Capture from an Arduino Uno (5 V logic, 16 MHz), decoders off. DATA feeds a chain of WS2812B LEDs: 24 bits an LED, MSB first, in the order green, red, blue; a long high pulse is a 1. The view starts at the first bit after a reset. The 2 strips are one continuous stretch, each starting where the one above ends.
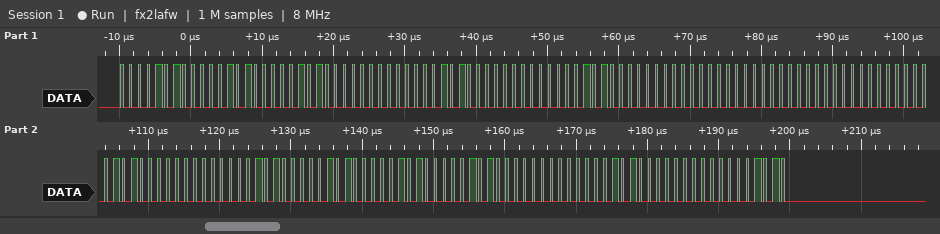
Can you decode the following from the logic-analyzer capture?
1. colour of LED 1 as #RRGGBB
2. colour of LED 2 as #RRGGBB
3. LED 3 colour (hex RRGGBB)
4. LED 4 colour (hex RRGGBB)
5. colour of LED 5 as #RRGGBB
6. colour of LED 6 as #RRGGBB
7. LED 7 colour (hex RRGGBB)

#0A0A0A
#0A0000
#000A00
#00000A
#0A000A
#0A0A00
#000A0A
